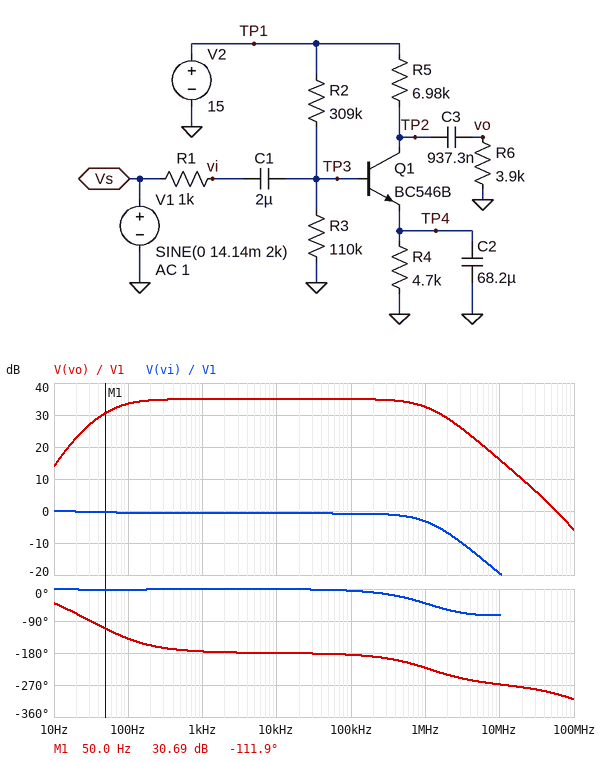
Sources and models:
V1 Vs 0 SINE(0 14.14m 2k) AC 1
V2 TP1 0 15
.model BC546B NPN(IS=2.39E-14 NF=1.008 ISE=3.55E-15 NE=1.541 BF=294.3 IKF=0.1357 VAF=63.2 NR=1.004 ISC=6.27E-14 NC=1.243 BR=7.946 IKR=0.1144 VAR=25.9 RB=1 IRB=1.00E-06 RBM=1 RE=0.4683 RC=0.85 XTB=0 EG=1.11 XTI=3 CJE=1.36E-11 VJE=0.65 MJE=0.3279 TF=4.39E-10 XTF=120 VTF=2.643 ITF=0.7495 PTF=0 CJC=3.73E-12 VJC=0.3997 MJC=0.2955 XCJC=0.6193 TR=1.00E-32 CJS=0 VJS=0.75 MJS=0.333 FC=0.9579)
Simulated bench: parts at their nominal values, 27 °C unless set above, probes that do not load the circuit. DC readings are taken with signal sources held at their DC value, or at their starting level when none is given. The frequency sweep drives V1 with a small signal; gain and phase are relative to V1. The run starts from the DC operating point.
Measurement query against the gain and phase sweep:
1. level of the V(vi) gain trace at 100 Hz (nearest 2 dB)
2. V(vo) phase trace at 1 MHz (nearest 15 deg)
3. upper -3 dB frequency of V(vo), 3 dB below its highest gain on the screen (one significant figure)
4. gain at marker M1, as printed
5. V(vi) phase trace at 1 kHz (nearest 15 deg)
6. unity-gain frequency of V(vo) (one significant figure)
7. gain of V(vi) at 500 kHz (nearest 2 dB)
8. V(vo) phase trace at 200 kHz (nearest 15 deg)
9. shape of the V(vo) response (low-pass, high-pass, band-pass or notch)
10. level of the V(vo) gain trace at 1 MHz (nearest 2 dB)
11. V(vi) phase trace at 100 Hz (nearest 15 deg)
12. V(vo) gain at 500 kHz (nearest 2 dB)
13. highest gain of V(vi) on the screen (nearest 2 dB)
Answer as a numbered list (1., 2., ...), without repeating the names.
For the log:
1. 0 dB
2. -225 deg
3. 1 MHz
4. 30.69 dB
5. 0 deg
6. 60 MHz
7. -2 dB
8. -195 deg
9. band-pass
10. 32 dB
11. 0 deg
12. 34 dB
13. 0 dB
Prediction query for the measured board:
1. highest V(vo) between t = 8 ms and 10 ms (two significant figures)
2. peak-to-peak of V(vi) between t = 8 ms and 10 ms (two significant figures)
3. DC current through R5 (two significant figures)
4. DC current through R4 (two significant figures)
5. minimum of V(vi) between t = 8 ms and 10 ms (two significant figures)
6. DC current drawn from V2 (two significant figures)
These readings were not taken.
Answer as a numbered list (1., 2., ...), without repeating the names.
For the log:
1. 700 mV
2. 26 mV
3. 670 µA
4. 670 µA
5. -13 mV
6. 700 µA
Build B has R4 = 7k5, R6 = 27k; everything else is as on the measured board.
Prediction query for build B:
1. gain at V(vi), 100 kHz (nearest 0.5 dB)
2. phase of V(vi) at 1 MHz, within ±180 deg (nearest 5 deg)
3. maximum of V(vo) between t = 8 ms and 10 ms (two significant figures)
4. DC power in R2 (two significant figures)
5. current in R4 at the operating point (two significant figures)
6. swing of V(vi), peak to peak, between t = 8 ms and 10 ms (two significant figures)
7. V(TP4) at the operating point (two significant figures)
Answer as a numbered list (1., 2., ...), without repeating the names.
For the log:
1. -0.5 dB
2. -45 deg
3. 1.0 V
4. 400 µW
5. 430 µA
6. 27 mV
7. 3.2 V
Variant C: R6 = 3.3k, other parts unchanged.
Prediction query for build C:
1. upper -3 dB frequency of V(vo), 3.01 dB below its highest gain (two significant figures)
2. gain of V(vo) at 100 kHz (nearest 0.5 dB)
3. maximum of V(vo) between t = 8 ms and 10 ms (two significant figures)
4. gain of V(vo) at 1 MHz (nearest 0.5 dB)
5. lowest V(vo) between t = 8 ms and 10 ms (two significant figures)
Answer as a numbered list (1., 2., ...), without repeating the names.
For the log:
1. 1.2 MHz
2. 34.0 dB
3. 630 mV
4. 32.0 dB
5. -760 mV
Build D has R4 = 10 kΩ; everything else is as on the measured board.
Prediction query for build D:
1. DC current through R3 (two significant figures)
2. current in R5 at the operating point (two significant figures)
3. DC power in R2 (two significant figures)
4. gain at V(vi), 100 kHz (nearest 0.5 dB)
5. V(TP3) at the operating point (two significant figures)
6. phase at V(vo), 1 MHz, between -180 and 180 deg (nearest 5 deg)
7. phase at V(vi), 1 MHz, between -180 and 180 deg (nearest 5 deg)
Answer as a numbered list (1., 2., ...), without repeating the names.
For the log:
1. 35 µA
2. 320 µA
3. 400 µW
4. -0.5 dB
5. 3.9 V
6. 150 deg
7. -25 deg
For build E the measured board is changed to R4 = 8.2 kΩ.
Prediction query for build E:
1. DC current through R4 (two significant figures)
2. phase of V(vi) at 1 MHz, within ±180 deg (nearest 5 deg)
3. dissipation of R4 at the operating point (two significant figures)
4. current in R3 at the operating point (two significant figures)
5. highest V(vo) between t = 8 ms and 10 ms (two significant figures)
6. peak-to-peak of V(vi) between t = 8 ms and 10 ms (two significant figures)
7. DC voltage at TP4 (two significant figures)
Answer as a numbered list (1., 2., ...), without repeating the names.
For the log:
1. 390 µA
2. -30 deg
3. 1.3 mW
4. 35 µA
5. 430 mV
6. 27 mV
7. 3.2 V
